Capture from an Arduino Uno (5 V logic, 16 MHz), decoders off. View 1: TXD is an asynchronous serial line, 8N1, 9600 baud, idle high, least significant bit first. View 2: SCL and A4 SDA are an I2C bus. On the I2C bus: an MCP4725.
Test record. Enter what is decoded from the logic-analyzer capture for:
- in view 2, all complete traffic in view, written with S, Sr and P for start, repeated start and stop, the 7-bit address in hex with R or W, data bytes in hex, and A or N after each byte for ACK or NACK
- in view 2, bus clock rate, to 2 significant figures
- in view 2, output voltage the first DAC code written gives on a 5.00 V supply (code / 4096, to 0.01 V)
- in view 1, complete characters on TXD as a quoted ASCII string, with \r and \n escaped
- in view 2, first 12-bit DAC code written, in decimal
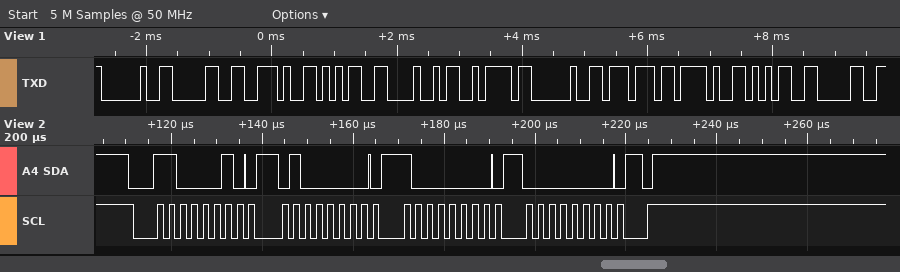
S 61W A 40 A 80 A 00 A P
400 kHz
2.50 V
" 0.5Hz w/50"
2048
